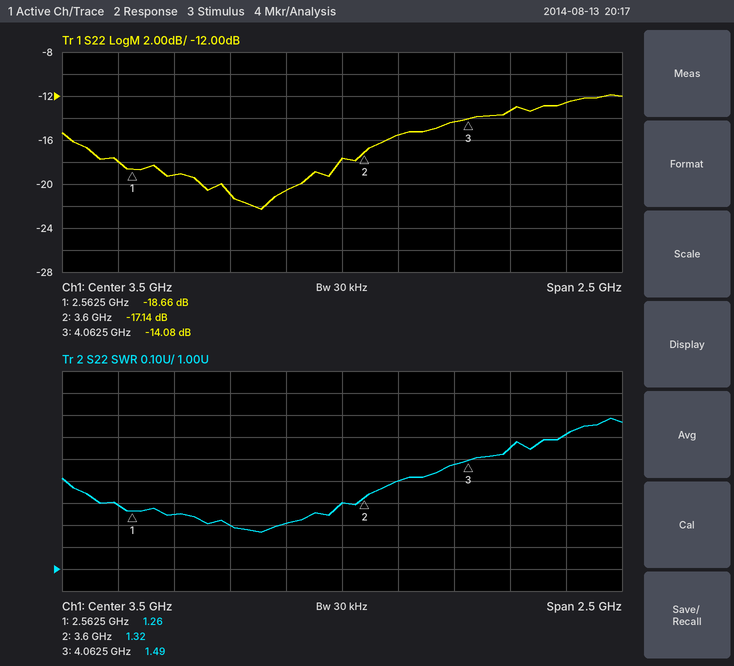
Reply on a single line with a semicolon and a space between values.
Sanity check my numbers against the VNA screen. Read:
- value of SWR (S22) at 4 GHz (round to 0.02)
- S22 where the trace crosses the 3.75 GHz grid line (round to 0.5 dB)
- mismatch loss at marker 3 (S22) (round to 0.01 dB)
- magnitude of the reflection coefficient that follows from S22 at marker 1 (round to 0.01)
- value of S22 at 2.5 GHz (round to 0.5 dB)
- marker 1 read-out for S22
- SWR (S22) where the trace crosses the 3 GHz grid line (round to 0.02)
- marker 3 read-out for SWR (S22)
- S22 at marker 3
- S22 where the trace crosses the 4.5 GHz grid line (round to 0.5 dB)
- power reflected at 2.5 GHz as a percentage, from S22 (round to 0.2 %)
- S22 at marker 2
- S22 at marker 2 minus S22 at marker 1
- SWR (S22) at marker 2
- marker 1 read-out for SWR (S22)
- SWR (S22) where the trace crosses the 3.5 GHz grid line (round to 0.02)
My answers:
1.48; -15.5 dB; 0.17 dB; 0.12; -18.0 dB; -18.66 dB; 1.20; 1.49; -14.08 dB; -12.5 dB; 1.6 %; -17.14 dB; 1.52 dB; 1.32; 1.26; 1.30
